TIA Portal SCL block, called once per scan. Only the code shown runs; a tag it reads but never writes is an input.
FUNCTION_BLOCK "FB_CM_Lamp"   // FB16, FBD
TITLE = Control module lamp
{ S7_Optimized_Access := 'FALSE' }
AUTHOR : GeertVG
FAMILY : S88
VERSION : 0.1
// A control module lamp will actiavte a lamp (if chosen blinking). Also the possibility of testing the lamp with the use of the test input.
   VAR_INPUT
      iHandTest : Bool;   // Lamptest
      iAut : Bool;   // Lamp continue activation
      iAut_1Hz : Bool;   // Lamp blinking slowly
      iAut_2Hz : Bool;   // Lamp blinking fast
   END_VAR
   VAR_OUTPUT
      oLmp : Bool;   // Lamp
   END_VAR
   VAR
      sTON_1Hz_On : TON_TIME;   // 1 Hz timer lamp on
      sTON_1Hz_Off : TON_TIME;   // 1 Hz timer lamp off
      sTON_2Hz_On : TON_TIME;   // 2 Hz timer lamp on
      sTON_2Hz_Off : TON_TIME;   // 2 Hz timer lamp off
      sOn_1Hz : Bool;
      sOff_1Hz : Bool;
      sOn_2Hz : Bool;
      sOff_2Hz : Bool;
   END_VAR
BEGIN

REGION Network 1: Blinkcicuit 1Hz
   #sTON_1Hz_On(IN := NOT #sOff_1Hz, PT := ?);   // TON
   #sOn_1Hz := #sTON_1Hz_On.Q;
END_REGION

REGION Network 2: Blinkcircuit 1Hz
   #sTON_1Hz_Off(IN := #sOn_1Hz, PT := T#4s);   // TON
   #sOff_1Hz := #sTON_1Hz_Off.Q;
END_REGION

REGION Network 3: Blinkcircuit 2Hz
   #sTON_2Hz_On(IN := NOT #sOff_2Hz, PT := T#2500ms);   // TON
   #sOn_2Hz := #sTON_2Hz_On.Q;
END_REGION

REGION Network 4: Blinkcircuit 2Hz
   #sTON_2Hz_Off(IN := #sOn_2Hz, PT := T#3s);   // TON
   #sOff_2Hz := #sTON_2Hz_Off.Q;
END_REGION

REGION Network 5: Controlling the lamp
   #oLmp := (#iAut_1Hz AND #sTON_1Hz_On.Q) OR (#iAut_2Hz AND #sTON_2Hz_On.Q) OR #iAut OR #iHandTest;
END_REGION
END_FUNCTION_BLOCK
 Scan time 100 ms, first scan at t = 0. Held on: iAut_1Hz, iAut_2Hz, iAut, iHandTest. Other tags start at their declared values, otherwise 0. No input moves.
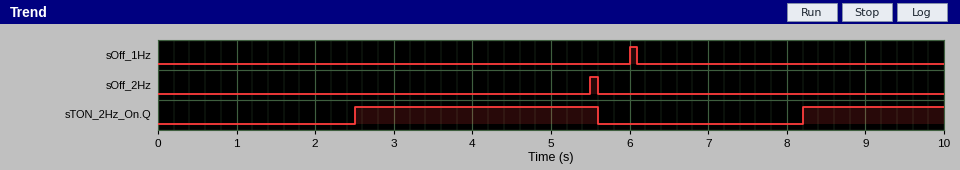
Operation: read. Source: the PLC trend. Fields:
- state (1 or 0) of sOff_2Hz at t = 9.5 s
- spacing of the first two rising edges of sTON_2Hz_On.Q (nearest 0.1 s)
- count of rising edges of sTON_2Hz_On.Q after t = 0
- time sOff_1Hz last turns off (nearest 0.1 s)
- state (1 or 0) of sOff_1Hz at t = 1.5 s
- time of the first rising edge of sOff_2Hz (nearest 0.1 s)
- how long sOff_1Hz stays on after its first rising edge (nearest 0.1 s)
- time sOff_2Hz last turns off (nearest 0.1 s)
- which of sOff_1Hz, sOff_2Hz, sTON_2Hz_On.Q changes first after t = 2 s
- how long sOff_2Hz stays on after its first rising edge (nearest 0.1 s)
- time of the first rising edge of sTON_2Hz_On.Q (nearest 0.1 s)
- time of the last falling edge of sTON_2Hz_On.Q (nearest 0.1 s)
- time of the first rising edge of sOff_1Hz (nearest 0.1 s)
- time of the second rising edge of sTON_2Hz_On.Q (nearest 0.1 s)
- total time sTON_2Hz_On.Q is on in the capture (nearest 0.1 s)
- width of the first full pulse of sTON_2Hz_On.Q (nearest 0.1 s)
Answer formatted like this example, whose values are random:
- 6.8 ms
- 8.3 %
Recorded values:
- 0
- 5.7 s
- 2
- 6.1 s
- 0
- 5.5 s
- 0.1 s
- 5.6 s
- sTON_2Hz_On.Q
- 0.1 s
- 2.5 s
- 5.6 s
- 6.0 s
- 8.2 s
- 4.9 s
- 3.1 s
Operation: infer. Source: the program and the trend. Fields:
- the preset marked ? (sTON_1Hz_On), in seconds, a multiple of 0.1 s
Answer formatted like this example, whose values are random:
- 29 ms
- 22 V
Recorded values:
- 2.0 s
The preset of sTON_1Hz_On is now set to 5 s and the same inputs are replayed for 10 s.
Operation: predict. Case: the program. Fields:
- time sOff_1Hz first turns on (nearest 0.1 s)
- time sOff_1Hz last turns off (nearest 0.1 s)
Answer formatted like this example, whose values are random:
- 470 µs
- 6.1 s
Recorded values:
- 9.0 s
- 9.1 s
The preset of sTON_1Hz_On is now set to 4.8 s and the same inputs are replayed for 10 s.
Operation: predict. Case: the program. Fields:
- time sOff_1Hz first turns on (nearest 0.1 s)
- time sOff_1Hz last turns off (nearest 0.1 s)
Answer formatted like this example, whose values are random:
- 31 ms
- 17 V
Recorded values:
- 8.8 s
- 8.9 s
